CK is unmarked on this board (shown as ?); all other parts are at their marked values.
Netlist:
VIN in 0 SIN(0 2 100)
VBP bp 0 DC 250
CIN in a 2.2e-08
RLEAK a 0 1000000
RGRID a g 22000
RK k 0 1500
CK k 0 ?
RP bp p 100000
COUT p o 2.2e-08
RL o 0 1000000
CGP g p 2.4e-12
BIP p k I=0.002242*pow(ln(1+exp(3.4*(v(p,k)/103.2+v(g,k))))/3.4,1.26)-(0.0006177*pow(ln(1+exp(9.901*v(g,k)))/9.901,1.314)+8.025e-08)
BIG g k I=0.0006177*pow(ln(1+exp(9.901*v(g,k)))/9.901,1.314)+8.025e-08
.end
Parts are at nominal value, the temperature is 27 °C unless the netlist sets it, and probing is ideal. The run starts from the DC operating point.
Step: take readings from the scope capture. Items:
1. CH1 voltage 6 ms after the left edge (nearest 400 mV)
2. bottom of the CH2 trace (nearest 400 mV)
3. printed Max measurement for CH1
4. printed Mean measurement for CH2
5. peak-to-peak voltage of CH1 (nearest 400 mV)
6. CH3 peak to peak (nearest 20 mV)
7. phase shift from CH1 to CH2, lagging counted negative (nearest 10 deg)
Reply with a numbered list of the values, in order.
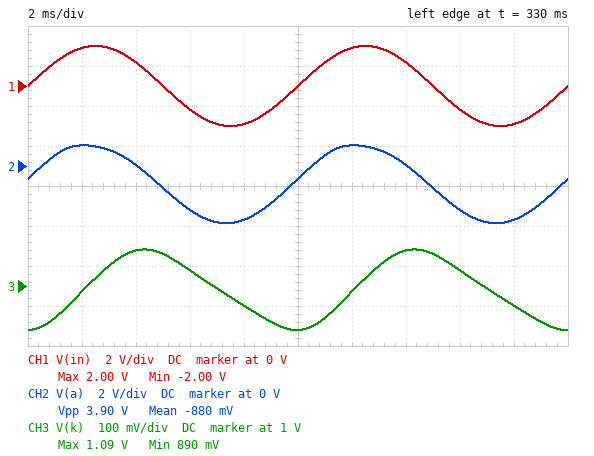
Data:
1. -1.2 V
2. -2.8 V
3. 2.00 V
4. -880 mV
5. 4.0 V
6. 200 mV
7. 10 deg
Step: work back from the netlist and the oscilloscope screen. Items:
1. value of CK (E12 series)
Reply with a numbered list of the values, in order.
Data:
1. 15 µF
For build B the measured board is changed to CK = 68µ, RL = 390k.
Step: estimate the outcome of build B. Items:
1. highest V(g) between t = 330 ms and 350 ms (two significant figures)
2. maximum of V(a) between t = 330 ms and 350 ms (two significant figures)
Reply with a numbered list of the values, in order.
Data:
1. 920 mV
2. 1.1 V
